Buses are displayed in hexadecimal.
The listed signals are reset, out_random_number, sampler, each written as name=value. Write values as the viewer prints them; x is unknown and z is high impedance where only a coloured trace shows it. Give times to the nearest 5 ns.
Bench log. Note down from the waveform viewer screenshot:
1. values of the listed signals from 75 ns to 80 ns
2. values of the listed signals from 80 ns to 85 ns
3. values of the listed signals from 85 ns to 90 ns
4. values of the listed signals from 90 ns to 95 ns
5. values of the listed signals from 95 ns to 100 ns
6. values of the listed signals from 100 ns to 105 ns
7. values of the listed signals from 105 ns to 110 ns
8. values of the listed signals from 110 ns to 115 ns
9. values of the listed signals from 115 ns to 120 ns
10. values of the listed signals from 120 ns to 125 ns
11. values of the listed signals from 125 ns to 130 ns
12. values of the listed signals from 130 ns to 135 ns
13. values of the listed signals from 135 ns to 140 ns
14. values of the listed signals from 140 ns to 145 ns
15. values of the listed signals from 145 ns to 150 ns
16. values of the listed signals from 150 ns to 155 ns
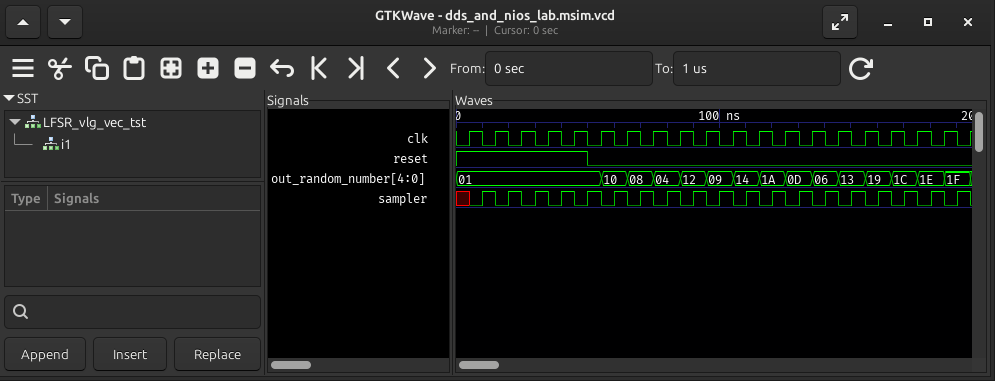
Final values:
reset=0, out_random_number=04, sampler=0
reset=0, out_random_number=04, sampler=1
reset=0, out_random_number=12, sampler=0
reset=0, out_random_number=12, sampler=1
reset=0, out_random_number=09, sampler=0
reset=0, out_random_number=09, sampler=1
reset=0, out_random_number=14, sampler=0
reset=0, out_random_number=14, sampler=1
reset=0, out_random_number=1A, sampler=0
reset=0, out_random_number=1A, sampler=1
reset=0, out_random_number=0D, sampler=0
reset=0, out_random_number=0D, sampler=1
reset=0, out_random_number=06, sampler=0
reset=0, out_random_number=06, sampler=1
reset=0, out_random_number=13, sampler=0
reset=0, out_random_number=13, sampler=1
